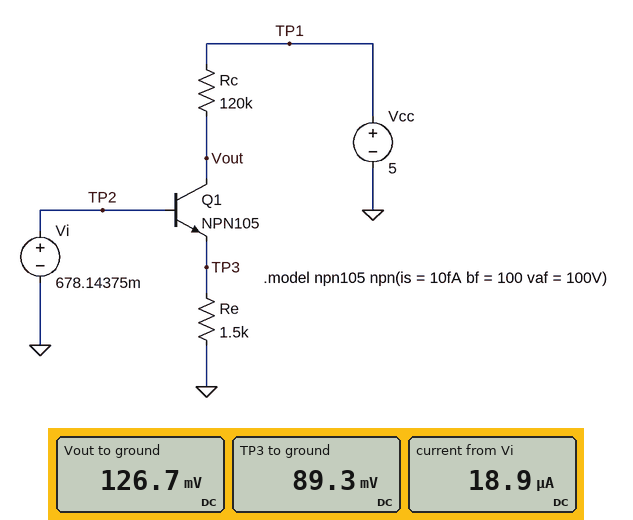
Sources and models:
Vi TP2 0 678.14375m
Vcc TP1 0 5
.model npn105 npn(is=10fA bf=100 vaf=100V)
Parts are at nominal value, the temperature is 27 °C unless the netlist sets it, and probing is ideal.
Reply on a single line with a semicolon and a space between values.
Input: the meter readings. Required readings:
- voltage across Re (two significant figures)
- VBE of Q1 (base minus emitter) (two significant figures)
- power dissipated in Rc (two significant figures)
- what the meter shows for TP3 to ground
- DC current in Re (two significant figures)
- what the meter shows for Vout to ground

89 mV; 590 mV; 200 µW; 89.3 mV; 60 µA; 126.7 mV
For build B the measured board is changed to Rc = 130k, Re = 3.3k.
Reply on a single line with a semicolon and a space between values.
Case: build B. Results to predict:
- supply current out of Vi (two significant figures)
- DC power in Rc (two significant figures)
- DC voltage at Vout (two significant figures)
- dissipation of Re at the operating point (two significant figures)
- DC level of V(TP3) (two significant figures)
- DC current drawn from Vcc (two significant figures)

330 nA; 140 µW; 670 mV; 3.7 µW; 110 mV; 33 µA
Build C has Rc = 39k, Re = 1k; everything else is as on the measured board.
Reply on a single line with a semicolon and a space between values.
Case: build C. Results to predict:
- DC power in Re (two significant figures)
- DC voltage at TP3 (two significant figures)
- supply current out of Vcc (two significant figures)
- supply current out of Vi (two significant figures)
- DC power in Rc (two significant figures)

7.5 µW; 87 mV; 86 µA; 850 nA; 290 µW
